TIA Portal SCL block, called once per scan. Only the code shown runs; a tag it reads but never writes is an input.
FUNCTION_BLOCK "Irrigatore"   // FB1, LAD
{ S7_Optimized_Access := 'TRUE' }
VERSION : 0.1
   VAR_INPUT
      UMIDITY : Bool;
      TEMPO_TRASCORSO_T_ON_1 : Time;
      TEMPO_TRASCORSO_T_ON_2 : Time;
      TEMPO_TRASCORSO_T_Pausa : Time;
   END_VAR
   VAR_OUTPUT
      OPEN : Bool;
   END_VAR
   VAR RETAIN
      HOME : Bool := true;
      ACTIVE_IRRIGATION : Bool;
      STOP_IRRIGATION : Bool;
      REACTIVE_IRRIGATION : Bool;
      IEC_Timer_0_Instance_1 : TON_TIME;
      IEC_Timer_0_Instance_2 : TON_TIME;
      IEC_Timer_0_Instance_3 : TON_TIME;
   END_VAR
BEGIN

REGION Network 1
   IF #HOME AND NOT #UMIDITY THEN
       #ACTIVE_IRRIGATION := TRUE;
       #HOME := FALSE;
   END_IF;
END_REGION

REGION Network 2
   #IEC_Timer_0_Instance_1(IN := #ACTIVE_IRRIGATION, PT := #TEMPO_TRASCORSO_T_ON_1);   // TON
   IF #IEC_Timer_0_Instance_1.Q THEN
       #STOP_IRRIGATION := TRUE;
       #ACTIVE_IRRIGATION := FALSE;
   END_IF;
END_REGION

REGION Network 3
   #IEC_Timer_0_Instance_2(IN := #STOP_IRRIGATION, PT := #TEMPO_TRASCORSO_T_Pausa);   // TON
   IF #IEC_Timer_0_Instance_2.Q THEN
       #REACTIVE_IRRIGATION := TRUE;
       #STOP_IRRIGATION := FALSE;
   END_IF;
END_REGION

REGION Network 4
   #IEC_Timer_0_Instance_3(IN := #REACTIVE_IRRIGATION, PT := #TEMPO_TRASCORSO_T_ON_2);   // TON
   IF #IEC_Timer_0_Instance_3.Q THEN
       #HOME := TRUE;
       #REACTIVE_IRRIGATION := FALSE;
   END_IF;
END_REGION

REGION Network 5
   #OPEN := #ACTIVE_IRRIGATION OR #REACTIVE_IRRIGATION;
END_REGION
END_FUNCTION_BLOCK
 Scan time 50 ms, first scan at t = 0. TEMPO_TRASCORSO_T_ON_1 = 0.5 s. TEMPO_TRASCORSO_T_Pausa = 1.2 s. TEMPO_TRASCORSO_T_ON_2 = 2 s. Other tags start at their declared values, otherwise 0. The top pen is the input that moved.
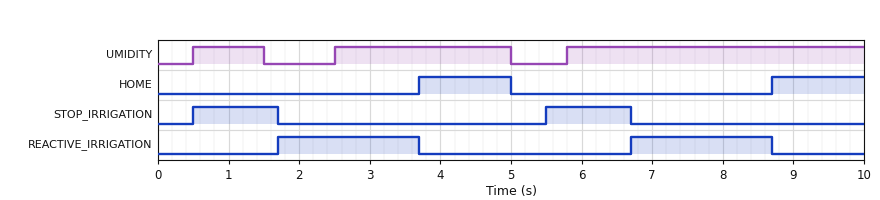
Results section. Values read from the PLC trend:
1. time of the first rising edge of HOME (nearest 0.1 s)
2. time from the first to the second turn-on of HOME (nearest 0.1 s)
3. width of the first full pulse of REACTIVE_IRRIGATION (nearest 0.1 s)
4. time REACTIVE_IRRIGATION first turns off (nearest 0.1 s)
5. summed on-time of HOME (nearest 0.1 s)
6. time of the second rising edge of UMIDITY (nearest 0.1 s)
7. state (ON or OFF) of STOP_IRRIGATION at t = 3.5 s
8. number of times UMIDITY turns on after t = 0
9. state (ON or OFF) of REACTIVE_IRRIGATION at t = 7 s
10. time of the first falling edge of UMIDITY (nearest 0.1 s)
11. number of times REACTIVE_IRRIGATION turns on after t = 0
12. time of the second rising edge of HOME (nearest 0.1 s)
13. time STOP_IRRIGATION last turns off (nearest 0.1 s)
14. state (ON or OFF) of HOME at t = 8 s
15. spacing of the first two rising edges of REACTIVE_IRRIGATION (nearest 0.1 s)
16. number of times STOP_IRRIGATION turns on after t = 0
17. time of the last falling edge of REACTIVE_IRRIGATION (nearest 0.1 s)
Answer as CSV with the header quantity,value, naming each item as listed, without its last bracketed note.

quantity,value
time of the first rising edge of HOME,3.7 s
time from the first to the second turn-on of HOME,5.0 s
width of the first full pulse of REACTIVE_IRRIGATION,2.0 s
time REACTIVE_IRRIGATION first turns off,3.7 s
summed on-time of HOME,2.6 s
time of the second rising edge of UMIDITY,2.5 s
state (ON or OFF) of STOP_IRRIGATION at t = 3.5 s,OFF
number of times UMIDITY turns on after t = 0,3
state (ON or OFF) of REACTIVE_IRRIGATION at t = 7 s,ON
time of the first falling edge of UMIDITY,1.5 s
number of times REACTIVE_IRRIGATION turns on after t = 0,2
time of the second rising edge of HOME,8.7 s
time STOP_IRRIGATION last turns off,6.7 s
state (ON or OFF) of HOME at t = 8 s,OFF
spacing of the first two rising edges of REACTIVE_IRRIGATION,5.0 s
number of times STOP_IRRIGATION turns on after t = 0,2
time of the last falling edge of REACTIVE_IRRIGATION,8.7 s
